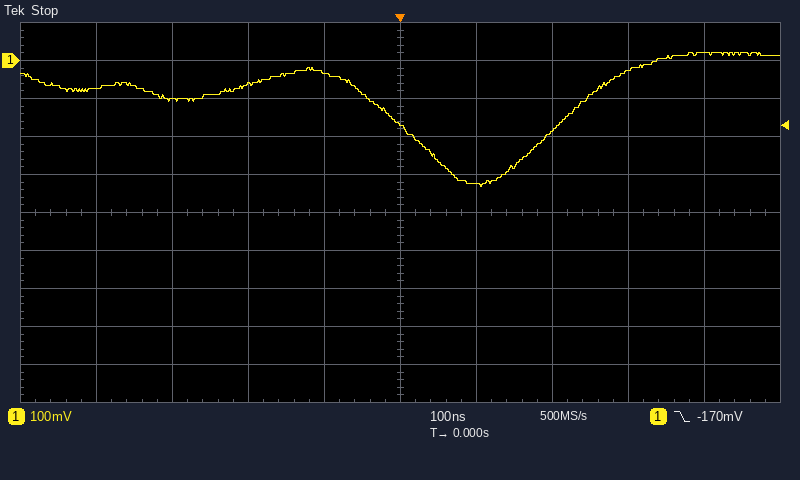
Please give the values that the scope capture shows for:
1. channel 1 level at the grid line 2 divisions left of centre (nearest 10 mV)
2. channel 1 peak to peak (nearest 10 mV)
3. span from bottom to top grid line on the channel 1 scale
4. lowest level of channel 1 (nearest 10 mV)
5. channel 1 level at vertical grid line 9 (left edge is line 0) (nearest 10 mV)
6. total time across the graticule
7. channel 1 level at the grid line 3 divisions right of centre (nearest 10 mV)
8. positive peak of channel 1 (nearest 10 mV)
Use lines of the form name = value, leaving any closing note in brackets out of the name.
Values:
channel 1 level at the grid line 2 divisions left of centre = -60 mV
channel 1 peak to peak = 350 mV
span from bottom to top grid line on the channel 1 scale = 1 V
lowest level of channel 1 = -330 mV
channel 1 level at vertical grid line 9 (left edge is line 0) = 20 mV
total time across the graticule = 1 µs
channel 1 level at the grid line 3 divisions right of centre = -30 mV
positive peak of channel 1 = 20 mV
